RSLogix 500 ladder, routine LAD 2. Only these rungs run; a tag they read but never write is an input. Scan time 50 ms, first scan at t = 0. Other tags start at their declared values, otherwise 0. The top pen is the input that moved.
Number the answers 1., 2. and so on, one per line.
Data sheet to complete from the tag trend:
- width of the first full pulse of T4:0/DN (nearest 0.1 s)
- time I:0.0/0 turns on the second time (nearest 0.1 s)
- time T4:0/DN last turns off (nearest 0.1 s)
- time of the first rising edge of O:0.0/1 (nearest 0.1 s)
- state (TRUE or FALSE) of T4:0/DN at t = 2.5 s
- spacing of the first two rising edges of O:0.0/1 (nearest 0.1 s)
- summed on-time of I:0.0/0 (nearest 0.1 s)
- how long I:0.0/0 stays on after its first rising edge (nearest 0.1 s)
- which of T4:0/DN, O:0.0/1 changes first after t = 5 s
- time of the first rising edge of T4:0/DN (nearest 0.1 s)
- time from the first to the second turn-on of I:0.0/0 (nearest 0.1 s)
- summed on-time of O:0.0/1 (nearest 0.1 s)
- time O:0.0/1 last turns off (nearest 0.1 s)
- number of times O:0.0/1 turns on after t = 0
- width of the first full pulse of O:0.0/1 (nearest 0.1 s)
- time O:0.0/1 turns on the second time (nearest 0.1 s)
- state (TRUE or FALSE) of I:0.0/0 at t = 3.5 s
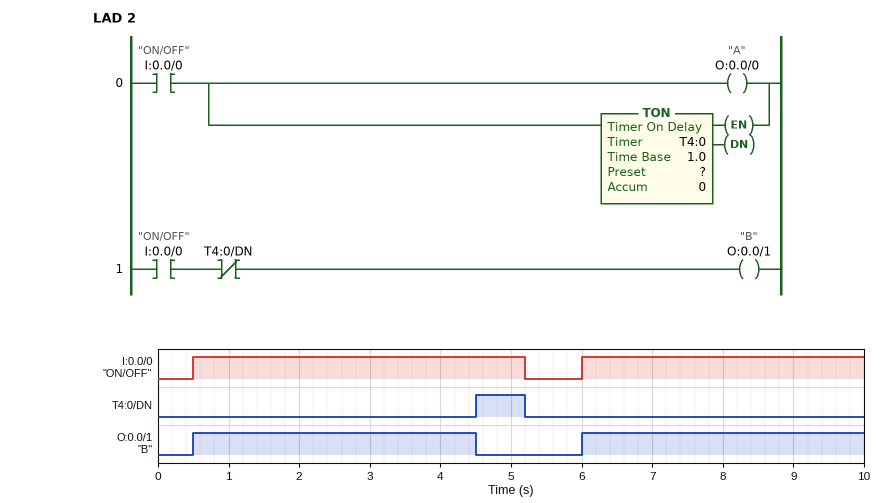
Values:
1. 0.7 s
2. 6.0 s
3. 5.2 s
4. 0.5 s
5. FALSE
6. 5.5 s
7. 8.7 s
8. 4.7 s
9. T4:0/DN
10. 4.5 s
11. 5.5 s
12. 8.0 s
13. 4.5 s
14. 2
15. 4.0 s
16. 6.0 s
17. TRUE
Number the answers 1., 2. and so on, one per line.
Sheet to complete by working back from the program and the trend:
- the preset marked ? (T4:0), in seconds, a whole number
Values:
1. 4 s
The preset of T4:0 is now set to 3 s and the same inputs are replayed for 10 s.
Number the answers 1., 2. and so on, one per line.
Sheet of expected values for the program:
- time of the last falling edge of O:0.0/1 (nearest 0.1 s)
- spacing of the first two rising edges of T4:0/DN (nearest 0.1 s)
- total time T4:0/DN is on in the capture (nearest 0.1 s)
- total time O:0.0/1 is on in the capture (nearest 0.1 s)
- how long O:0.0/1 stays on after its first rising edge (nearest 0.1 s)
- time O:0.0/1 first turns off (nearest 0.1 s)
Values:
1. 9.0 s
2. 5.5 s
3. 2.7 s
4. 6.0 s
5. 3.0 s
6. 3.5 s
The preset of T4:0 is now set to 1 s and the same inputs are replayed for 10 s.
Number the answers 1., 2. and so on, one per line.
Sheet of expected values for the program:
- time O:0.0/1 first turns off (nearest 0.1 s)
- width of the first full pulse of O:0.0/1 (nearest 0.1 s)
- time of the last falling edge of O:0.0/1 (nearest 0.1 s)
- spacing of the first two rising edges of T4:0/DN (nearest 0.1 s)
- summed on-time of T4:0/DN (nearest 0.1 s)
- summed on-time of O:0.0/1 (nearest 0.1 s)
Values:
1. 1.5 s
2. 1.0 s
3. 7.0 s
4. 5.5 s
5. 6.7 s
6. 2.0 s
